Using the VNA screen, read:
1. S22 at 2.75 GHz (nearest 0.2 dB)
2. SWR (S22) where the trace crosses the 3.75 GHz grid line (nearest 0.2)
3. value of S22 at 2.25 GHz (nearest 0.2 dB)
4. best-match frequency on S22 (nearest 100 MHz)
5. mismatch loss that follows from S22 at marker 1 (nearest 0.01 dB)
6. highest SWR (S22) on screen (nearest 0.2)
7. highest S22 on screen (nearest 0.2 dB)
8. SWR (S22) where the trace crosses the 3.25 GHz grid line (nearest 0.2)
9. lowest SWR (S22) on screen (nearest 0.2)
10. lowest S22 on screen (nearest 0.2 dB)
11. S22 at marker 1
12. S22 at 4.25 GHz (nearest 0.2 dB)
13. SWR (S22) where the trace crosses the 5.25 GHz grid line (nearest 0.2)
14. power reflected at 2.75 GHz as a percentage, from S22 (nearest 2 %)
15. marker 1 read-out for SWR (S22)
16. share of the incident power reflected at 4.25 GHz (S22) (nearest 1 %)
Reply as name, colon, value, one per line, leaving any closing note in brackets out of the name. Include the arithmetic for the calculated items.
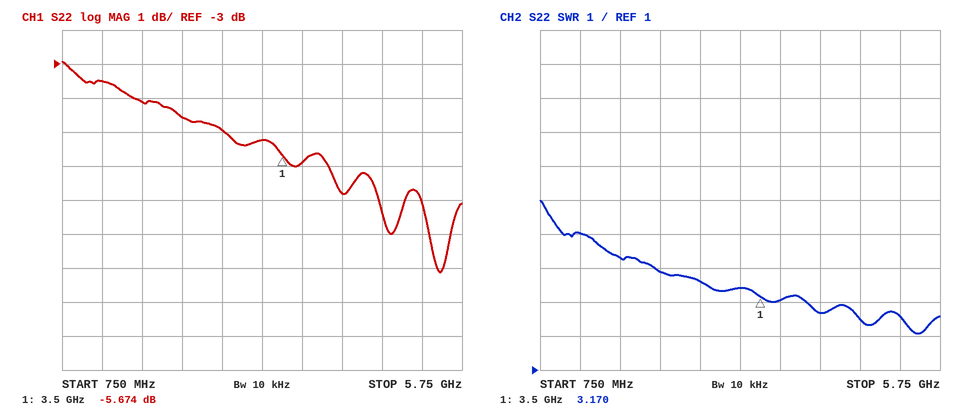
S22 at 2.75 GHz: -5.0 dB
SWR (S22) where the trace crosses the 3.75 GHz grid line: 3.0
value of S22 at 2.25 GHz: -4.6 dB
best-match frequency on S22: 5.5 GHz
mismatch loss that follows from S22 at marker 1: −10 log10(1 − 10^(-5.674/10)) ≈ 1.37 dB
highest SWR (S22) on screen: 6.0
highest S22 on screen: -3.0 dB
SWR (S22) where the trace crosses the 3.25 GHz grid line: 3.4
lowest SWR (S22) on screen: 2.0
lowest S22 on screen: -9.2 dB
S22 at marker 1: -5.674 dB
S22 at 4.25 GHz: -6.8 dB
SWR (S22) where the trace crosses the 5.25 GHz grid line: 2.6
power reflected at 2.75 GHz as a percentage, from S22: 10^(-5/10) ≈ 32 %
marker 1 read-out for SWR: 3.170
share of the incident power reflected at 4.25 GHz (S22): 10^(-6.8/10) ≈ 21 %
